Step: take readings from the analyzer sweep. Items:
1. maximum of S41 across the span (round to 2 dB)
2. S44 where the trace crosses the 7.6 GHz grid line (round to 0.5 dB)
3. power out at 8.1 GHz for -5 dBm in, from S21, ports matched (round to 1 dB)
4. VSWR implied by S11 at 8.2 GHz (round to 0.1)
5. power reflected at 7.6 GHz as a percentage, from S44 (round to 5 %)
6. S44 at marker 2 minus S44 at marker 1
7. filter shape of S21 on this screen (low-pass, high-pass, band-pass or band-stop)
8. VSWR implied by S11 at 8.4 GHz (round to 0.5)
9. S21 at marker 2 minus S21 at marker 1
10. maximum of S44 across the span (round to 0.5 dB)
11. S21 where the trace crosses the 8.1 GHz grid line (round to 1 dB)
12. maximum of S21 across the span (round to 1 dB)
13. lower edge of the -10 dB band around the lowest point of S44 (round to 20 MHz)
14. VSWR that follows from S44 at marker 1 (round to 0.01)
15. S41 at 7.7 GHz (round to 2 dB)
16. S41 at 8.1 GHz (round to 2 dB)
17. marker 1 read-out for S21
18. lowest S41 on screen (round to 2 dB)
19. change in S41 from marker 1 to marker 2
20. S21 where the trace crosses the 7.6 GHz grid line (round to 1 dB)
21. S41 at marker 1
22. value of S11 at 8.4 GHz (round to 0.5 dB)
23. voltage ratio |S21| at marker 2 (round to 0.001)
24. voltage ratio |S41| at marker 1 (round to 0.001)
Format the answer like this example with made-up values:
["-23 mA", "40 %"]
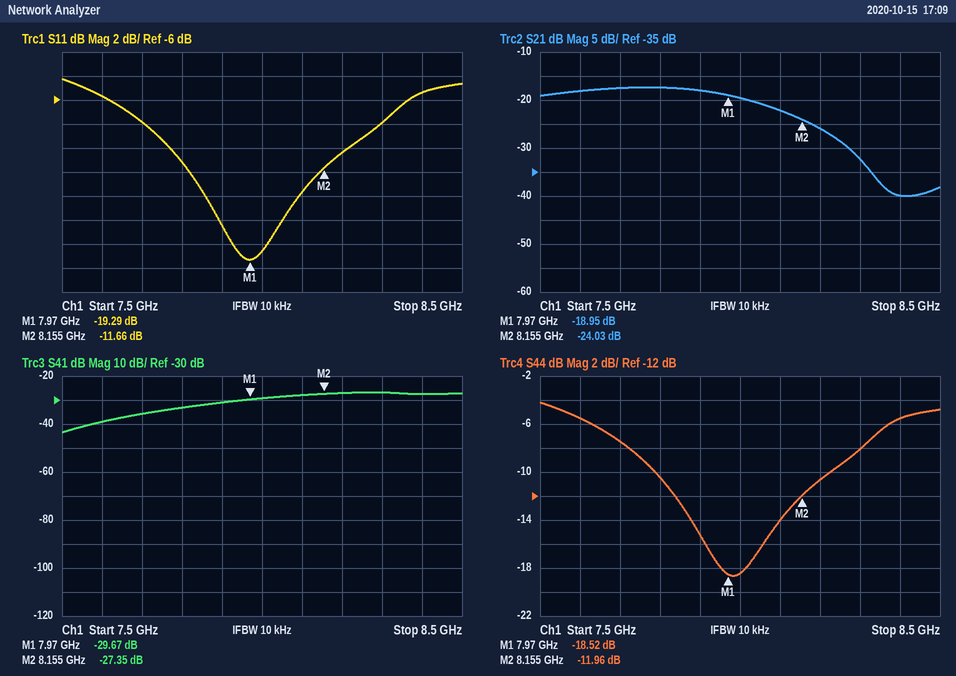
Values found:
["-26 dB", "-5.5 dB", "-27 dBm", "1.9", "30 %", "6.56 dB", "low-pass", "3.5", "-5.08 dB", "-4.0 dB", "-22 dB", "-17 dB", "7.78 GHz", "1.27", "-36 dB", "-28 dB", "-18.95 dB", "-44 dB", "2.32 dB", "-18 dB", "-29.67 dB", "-5.5 dB", "0.063", "0.033"]
